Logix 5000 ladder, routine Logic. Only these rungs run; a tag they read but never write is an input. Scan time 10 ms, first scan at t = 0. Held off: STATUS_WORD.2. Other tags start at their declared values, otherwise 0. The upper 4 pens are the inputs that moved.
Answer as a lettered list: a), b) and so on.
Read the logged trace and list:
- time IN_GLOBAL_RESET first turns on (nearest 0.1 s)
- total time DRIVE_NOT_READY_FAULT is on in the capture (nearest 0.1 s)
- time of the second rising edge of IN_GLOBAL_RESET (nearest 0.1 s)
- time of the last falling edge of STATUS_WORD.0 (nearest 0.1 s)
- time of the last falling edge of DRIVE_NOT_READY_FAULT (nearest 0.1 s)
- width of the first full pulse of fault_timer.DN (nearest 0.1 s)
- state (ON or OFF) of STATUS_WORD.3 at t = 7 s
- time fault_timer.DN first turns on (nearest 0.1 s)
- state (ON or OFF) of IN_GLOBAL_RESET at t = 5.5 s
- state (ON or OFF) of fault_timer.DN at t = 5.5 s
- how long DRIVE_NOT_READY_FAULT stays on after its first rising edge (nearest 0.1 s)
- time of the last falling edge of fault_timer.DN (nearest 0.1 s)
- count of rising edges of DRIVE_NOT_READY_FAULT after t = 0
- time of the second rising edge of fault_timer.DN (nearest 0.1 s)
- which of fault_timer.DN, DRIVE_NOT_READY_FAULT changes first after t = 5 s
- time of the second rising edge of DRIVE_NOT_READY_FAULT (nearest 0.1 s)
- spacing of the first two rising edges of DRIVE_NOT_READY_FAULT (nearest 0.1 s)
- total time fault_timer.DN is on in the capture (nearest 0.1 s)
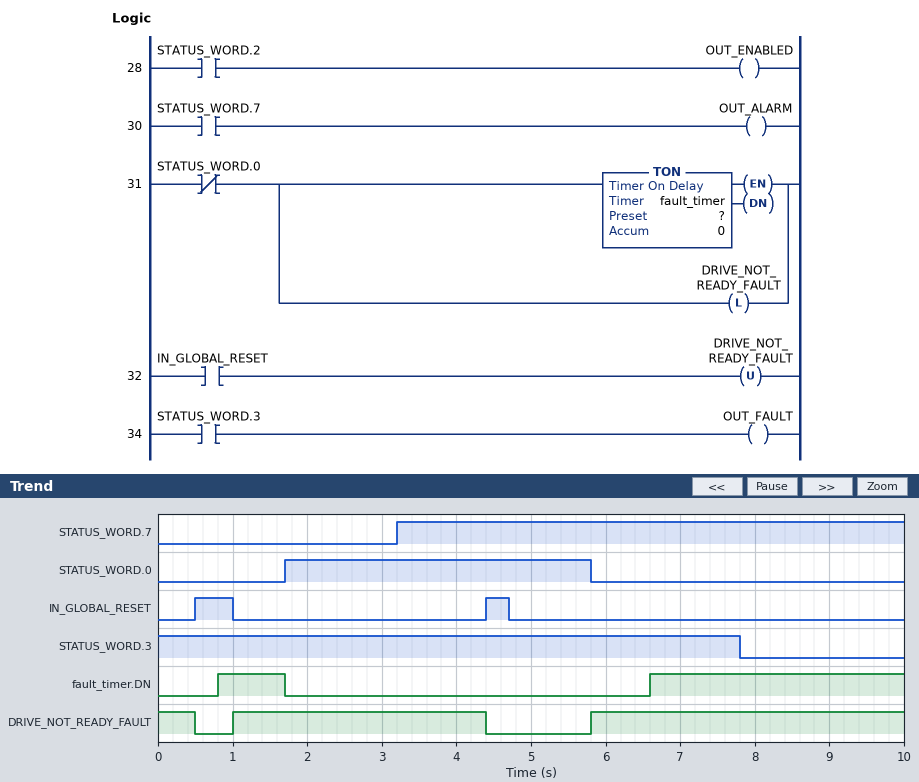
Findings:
a) 0.5 s
b) 8.1 s
c) 4.4 s
d) 5.8 s
e) 4.4 s
f) 0.9 s
g) ON
h) 0.8 s
i) OFF
j) OFF
k) 3.4 s
l) 1.7 s
m) 2
n) 6.6 s
o) DRIVE_NOT_READY_FAULT
p) 5.8 s
q) 4.8 s
r) 4.3 s
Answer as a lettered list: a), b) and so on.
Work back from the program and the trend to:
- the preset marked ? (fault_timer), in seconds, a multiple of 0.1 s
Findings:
a) 0.8 s
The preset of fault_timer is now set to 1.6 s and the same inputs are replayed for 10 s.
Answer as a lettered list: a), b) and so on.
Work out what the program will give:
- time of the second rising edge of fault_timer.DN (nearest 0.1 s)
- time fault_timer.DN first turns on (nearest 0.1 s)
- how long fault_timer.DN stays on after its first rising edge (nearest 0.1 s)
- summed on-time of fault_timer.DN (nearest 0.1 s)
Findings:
a) 7.4 s
b) 1.6 s
c) 0.1 s
d) 2.7 s
